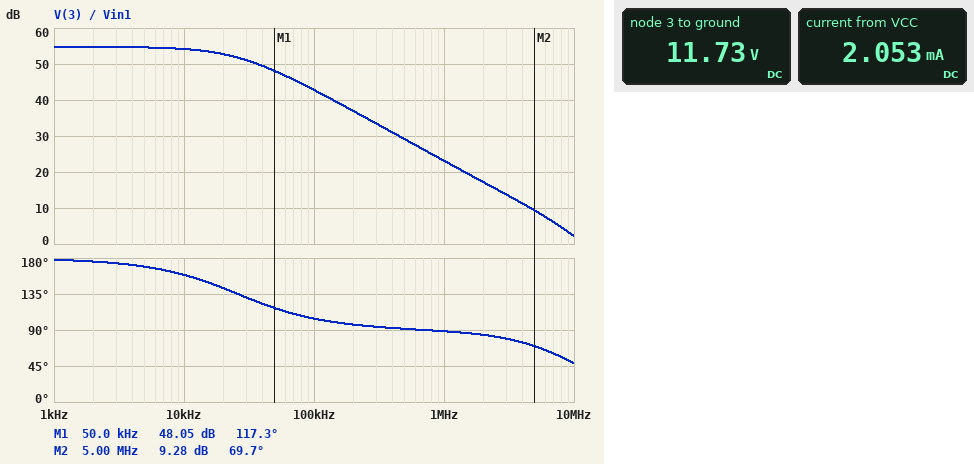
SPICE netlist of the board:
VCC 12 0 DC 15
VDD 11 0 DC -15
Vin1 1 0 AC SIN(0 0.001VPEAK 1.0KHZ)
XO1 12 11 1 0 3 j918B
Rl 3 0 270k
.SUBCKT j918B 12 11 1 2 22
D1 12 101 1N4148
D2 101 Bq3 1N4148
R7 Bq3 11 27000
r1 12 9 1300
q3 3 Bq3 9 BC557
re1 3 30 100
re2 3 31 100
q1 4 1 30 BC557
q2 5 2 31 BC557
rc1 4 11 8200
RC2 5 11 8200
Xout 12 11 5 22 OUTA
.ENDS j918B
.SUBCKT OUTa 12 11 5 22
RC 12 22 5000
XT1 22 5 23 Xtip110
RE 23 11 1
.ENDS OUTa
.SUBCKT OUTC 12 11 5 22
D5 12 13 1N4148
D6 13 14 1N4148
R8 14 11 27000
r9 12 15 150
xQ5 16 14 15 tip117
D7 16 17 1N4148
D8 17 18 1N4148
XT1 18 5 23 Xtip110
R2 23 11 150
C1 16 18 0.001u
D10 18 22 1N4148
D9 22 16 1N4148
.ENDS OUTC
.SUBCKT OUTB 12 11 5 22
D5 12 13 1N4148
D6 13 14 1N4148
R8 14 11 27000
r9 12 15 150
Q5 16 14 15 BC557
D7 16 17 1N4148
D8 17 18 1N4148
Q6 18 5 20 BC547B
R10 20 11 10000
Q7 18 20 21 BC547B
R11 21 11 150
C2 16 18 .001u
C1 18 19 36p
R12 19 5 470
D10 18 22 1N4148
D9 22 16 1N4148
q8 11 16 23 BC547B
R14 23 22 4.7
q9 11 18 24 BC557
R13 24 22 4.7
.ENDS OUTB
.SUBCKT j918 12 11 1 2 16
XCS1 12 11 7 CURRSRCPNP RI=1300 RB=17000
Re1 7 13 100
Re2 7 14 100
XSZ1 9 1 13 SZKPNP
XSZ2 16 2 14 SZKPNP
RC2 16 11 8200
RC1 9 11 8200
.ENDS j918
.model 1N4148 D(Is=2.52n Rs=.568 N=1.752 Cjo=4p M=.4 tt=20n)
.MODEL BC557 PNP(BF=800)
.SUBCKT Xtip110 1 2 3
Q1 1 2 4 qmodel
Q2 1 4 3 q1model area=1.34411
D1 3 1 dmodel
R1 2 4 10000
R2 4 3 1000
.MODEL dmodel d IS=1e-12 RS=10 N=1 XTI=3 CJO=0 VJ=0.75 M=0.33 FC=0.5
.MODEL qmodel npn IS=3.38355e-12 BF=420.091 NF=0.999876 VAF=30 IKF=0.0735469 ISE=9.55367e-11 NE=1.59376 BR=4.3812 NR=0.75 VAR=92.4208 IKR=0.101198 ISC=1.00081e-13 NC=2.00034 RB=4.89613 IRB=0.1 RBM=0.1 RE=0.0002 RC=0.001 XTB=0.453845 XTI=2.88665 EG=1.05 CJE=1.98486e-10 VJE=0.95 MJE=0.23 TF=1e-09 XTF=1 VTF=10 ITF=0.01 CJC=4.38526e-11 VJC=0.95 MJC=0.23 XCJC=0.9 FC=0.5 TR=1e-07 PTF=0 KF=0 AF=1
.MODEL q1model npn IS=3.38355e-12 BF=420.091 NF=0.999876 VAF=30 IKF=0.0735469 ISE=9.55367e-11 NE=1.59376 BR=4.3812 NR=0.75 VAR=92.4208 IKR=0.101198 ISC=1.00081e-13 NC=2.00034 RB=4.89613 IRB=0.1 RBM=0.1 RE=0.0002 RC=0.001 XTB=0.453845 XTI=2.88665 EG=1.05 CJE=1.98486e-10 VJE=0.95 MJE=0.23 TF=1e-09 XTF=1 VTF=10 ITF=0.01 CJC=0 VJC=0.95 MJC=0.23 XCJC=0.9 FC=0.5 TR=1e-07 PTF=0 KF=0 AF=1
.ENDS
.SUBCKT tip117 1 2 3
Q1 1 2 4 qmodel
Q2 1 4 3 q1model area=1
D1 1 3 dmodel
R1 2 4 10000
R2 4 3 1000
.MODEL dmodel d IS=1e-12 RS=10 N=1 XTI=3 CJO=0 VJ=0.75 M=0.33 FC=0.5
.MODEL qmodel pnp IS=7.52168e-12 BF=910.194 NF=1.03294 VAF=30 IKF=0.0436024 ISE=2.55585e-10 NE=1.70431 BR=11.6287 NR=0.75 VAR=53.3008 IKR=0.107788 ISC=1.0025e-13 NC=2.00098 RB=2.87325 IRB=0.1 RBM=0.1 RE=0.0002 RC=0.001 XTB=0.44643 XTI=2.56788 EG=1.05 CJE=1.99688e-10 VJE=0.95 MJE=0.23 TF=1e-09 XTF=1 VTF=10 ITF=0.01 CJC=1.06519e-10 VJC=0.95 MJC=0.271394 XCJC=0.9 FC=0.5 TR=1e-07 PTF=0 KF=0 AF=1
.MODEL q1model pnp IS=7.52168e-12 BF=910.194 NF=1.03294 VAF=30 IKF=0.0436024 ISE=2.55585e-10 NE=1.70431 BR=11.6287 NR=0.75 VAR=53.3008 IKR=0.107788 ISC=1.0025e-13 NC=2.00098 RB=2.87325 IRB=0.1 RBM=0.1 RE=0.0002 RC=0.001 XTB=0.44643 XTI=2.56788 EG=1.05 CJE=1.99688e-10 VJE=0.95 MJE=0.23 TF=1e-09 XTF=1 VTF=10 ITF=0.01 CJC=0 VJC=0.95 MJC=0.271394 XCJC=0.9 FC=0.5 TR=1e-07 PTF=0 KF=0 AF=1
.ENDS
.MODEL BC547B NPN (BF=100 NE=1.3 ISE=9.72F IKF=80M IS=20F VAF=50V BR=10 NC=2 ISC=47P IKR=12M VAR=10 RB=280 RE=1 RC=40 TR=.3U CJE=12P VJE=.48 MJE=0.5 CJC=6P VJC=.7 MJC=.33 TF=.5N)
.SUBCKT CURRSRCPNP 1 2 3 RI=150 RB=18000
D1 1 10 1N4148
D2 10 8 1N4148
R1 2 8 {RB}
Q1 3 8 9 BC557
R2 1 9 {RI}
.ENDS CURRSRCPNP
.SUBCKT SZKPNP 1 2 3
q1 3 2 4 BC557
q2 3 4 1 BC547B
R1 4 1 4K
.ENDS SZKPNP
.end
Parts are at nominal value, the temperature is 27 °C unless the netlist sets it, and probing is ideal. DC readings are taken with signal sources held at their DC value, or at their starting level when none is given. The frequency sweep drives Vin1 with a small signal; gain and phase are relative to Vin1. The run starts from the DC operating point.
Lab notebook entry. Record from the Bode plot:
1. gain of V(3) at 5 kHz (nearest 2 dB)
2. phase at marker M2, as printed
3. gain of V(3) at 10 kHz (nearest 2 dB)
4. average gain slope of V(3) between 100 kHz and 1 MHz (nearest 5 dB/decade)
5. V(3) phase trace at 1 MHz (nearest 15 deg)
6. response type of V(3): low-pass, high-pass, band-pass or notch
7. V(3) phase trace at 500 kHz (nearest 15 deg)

54 dB
69.7 deg
54 dB
-20 dB/decade
90 deg
low-pass
90 deg
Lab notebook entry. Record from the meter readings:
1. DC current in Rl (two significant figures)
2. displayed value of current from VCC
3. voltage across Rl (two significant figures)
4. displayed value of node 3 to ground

43 µA
2.053 mA
12 V
11.73 V
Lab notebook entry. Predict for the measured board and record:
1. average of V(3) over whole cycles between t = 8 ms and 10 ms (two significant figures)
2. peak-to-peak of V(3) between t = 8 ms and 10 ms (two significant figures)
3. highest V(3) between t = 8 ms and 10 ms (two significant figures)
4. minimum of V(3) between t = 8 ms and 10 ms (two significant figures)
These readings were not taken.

12 V
1.1 V
12 V
11 V
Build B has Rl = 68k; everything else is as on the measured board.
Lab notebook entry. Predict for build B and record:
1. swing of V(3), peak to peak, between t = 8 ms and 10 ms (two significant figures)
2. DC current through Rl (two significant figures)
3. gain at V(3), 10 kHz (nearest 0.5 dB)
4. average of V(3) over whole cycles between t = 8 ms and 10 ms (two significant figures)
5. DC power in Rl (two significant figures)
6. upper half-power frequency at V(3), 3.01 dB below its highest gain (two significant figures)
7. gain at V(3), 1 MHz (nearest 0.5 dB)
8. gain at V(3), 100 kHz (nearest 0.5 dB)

1.0 V
160 µA
53.5 dB
11 V
1.8 mW
28 kHz
23.0 dB
42.5 dB
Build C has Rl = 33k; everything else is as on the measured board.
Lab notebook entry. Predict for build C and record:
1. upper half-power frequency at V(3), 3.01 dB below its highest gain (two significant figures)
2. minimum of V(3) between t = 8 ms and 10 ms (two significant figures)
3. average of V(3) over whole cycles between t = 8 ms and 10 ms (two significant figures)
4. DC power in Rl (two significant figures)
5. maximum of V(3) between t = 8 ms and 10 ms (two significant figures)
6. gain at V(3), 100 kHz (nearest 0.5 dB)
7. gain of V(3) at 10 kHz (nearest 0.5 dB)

31 kHz
9.9 V
10 V
3.3 mW
11 V
42.5 dB
52.5 dB
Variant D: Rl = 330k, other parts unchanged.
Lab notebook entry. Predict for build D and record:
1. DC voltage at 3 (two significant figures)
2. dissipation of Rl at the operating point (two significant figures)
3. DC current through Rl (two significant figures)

12 V
420 µW
36 µA
